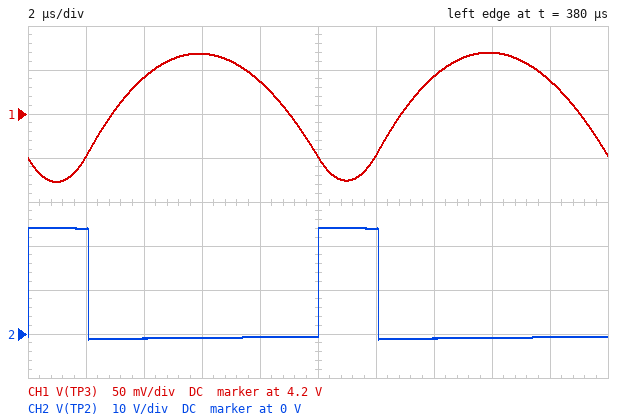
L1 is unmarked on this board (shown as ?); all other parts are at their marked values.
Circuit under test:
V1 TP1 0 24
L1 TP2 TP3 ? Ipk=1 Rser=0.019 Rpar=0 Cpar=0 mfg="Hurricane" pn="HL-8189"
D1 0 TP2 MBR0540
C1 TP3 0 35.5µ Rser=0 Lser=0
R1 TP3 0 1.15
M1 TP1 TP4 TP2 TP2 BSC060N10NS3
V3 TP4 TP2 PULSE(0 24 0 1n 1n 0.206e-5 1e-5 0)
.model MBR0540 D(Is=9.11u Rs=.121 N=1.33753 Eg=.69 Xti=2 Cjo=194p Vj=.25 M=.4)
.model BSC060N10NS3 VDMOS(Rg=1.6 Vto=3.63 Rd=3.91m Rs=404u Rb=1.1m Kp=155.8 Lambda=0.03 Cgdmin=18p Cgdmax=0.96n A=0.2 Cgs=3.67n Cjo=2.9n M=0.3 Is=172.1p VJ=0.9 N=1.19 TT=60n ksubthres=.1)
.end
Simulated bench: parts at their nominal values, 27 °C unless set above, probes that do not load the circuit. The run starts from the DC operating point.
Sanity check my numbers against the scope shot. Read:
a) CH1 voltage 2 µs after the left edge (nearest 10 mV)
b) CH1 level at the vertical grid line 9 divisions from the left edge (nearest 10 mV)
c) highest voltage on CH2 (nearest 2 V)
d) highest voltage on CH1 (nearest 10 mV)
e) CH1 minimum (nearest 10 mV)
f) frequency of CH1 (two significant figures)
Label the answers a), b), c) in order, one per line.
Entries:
a) 4.15 V
b) 4.24 V
c) 24 V
d) 4.27 V
e) 4.12 V
f) 100 kHz
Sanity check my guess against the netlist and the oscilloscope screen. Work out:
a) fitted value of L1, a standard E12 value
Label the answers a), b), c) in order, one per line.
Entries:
a) 10 µH
